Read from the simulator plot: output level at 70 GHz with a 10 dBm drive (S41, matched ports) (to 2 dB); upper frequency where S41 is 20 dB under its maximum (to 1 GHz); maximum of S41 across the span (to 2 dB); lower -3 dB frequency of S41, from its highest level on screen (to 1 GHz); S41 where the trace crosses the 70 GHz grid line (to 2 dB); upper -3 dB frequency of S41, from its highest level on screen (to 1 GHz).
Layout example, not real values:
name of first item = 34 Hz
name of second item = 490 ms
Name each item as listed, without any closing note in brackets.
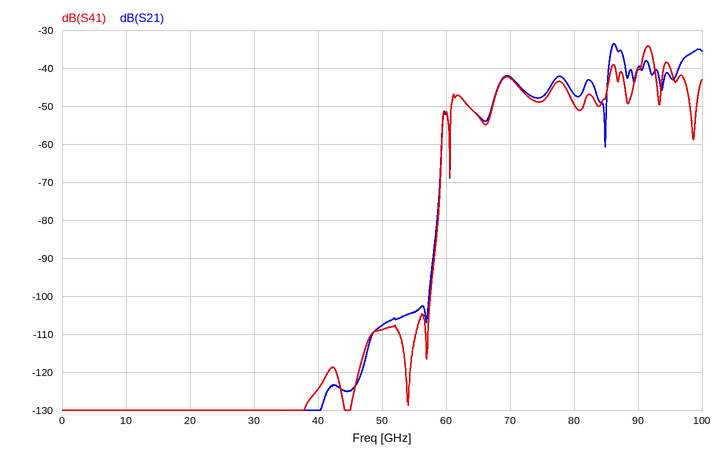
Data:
output level at 70 GHz with a 10 dBm drive (S41, matched ports) = -32 dBm
upper frequency where S41 is 20 dB under its maximum = 98 GHz
maximum of S41 across the span = -34 dB
lower -3 dB frequency of S41, from its highest level on screen = 91 GHz
S41 where the trace crosses the 70 GHz grid line = -42 dB
upper -3 dB frequency of S41, from its highest level on screen = 92 GHz
